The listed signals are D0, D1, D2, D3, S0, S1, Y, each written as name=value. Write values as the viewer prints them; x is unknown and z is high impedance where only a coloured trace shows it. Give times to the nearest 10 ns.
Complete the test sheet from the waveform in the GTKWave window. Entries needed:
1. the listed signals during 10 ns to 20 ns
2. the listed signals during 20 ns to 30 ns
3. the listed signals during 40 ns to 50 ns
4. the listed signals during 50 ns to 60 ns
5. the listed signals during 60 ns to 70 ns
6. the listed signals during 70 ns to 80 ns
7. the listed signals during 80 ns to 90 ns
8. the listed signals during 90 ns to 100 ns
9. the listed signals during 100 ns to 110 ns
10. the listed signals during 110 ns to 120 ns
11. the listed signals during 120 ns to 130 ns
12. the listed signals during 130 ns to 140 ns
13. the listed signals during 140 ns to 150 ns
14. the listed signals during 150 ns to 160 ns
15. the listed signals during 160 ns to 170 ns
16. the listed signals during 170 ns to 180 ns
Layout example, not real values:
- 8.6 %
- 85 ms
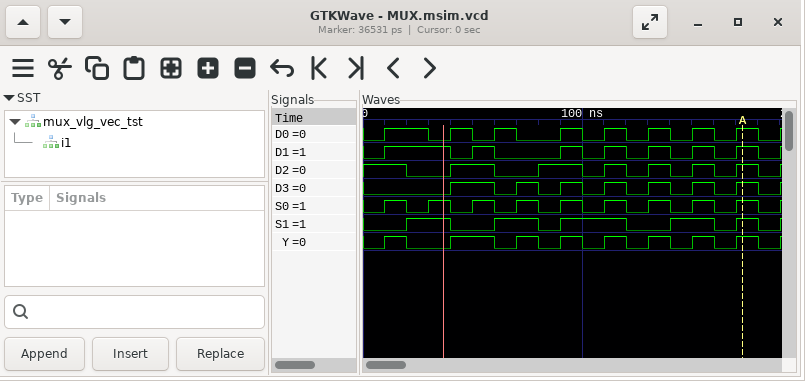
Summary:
- D0=1, D1=1, D2=1, D3=0, S0=1, S1=0, Y=1
- D0=1, D1=1, D2=0, D3=0, S0=0, S1=1, Y=0
- D0=1, D1=0, D2=1, D3=1, S0=0, S1=0, Y=1
- D0=0, D1=1, D2=1, D3=1, S0=1, S1=0, Y=1
- D0=1, D1=0, D2=0, D3=0, S0=0, S1=1, Y=0
- D0=0, D1=0, D2=0, D3=1, S0=1, S1=1, Y=1
- D0=0, D1=0, D2=1, D3=0, S0=0, S1=0, Y=0
- D0=1, D1=1, D2=1, D3=1, S0=1, S1=1, Y=1
- D0=0, D1=0, D2=0, D3=0, S0=0, S1=1, Y=0
- D0=1, D1=1, D2=1, D3=1, S0=1, S1=1, Y=1
- D0=0, D1=0, D2=0, D3=0, S0=0, S1=0, Y=0
- D0=1, D1=1, D2=1, D3=1, S0=1, S1=0, Y=1
- D0=0, D1=0, D2=0, D3=0, S0=0, S1=1, Y=0
- D0=1, D1=1, D2=1, D3=1, S0=1, S1=1, Y=1
- D0=0, D1=0, D2=0, D3=0, S0=0, S1=0, Y=0
- D0=1, D1=1, D2=1, D3=1, S0=1, S1=1, Y=1
